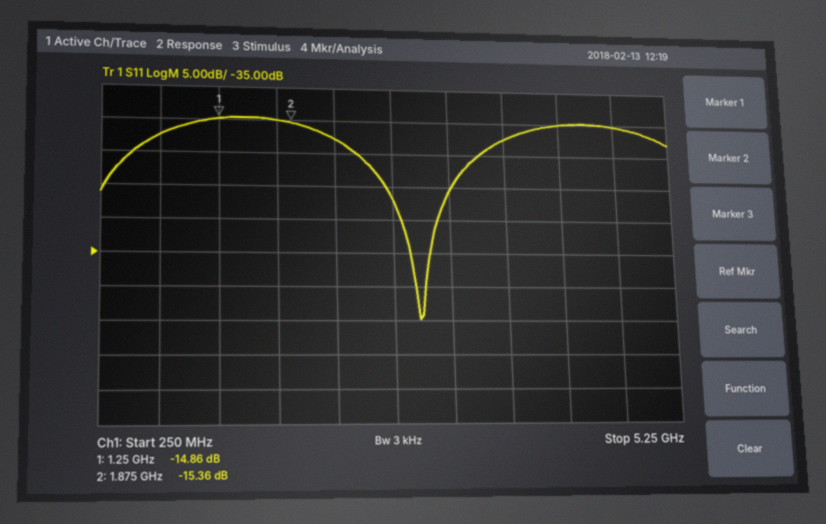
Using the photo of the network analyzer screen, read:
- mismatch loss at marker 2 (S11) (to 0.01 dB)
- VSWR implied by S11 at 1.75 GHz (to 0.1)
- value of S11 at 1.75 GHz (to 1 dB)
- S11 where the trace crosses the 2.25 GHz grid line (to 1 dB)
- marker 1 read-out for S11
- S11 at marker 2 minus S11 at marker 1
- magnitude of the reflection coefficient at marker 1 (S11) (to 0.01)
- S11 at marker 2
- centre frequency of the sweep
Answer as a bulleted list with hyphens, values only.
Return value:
- 0.13 dB
- 1.4
- -15 dB
- -18 dB
- -14.86 dB
- -0.50 dB
- 0.18
- -15.36 dB
- 2.75 GHz
